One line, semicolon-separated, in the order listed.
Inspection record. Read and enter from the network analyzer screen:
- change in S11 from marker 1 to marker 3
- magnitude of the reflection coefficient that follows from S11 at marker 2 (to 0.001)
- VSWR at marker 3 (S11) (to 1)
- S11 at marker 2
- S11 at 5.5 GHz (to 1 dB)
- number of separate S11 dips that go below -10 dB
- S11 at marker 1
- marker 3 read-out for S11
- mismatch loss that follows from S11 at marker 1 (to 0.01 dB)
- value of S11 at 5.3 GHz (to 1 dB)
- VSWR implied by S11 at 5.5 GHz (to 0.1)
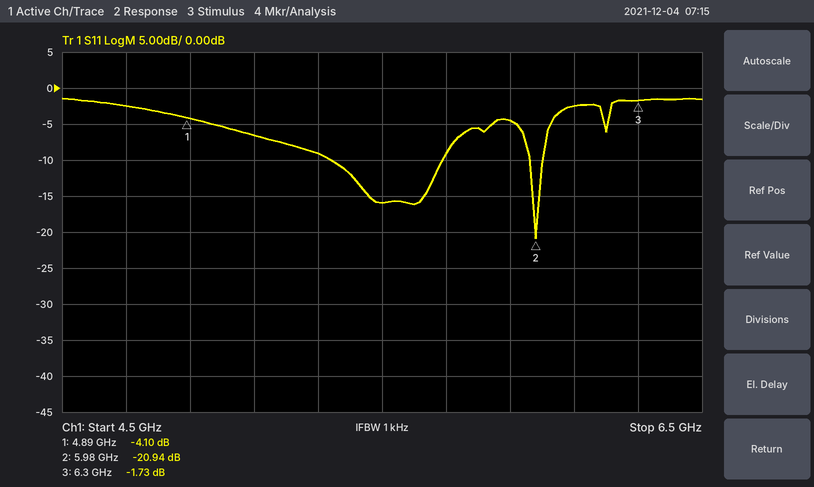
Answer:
2.37 dB; 0.090; 10; -20.94 dB; -16 dB; 2; -4.10 dB; -1.73 dB; 2.14 dB; -9 dB; 1.4
